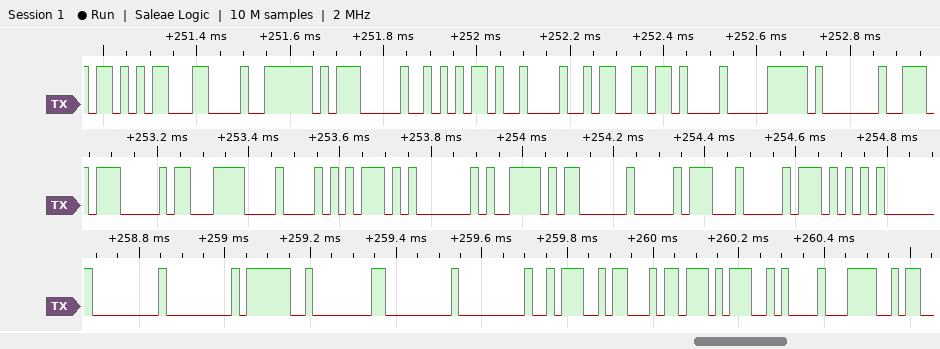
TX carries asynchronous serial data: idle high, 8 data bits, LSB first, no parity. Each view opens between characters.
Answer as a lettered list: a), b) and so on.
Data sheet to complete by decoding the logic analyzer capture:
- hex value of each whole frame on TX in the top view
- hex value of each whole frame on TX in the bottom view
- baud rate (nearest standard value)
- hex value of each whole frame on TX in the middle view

a) AB, 0C, 7E, 07, AA, 09, 9A, 0B, F0, 01
b) 00, 00, 3F, 80, 00, 00, 3A, A3, D7, 0A, 3C
c) 57600 baud
d) 07, E3, 08, 75, 01, 79, 03, D0, 04, 57
